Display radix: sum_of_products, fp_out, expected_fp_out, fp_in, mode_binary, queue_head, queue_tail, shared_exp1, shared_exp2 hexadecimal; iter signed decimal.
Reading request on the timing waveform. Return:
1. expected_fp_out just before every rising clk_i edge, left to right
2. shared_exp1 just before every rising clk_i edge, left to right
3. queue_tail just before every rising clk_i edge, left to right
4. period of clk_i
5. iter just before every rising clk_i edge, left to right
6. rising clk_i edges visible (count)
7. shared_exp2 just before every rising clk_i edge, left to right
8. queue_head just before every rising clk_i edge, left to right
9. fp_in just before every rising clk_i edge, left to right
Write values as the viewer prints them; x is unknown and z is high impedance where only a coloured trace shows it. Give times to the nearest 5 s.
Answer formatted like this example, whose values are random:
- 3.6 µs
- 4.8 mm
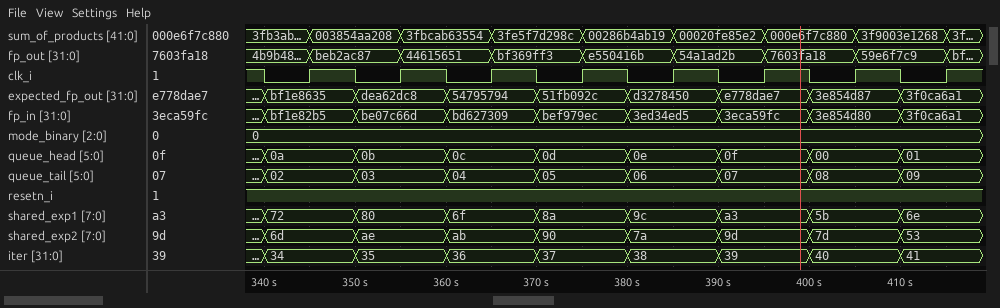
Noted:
- bf1e8635, dea62dc8, 54795794, 51fb092c, d3278450, e778dae7, 3e854d87, 3f0ca6a1
- 72, 80, 6f, 8a, 9c, a3, 5b, 6e
- 02, 03, 04, 05, 06, 07, 08, 09
- 10 s
- 34, 35, 36, 37, 38, 39, 40, 41
- 8
- 6d, ae, ab, 90, 7a, 9d, 7d, 53
- 0a, 0b, 0c, 0d, 0e, 0f, 00, 01
- bf1e82b5, be07c66d, bd627309, bef979ec, 3ed34ed5, 3eca59fc, 3e854d80, 3f0ca6a1
